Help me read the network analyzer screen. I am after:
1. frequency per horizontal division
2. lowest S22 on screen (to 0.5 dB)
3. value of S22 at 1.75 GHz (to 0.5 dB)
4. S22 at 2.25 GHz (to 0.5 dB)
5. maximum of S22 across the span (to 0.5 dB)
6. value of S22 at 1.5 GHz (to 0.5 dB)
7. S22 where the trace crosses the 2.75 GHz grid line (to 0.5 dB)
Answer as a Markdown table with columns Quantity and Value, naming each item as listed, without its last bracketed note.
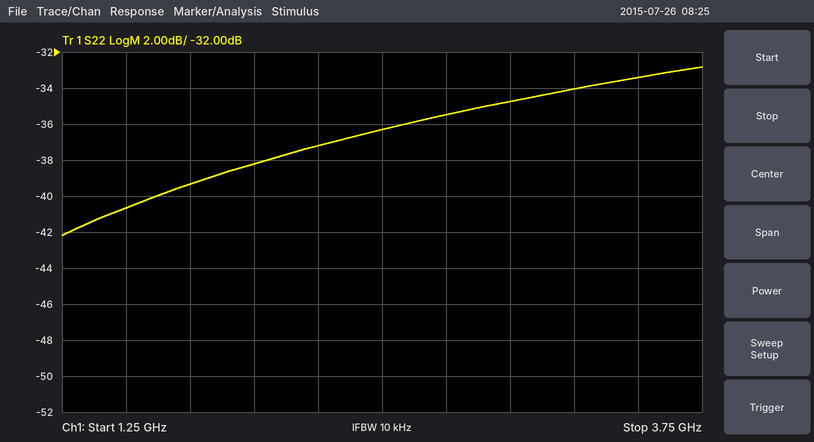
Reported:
| Quantity | Value |
|---|---|
| frequency per horizontal division | 250 MHz |
| lowest S22 on screen | -42.0 dB |
| value of S22 at 1.75 GHz | -39.5 dB |
| S22 at 2.25 GHz | -37.0 dB |
| maximum of S22 across the span | -33.0 dB |
| value of S22 at 1.5 GHz | -40.5 dB |
| S22 where the trace crosses the 2.75 GHz grid line | -35.5 dB |
